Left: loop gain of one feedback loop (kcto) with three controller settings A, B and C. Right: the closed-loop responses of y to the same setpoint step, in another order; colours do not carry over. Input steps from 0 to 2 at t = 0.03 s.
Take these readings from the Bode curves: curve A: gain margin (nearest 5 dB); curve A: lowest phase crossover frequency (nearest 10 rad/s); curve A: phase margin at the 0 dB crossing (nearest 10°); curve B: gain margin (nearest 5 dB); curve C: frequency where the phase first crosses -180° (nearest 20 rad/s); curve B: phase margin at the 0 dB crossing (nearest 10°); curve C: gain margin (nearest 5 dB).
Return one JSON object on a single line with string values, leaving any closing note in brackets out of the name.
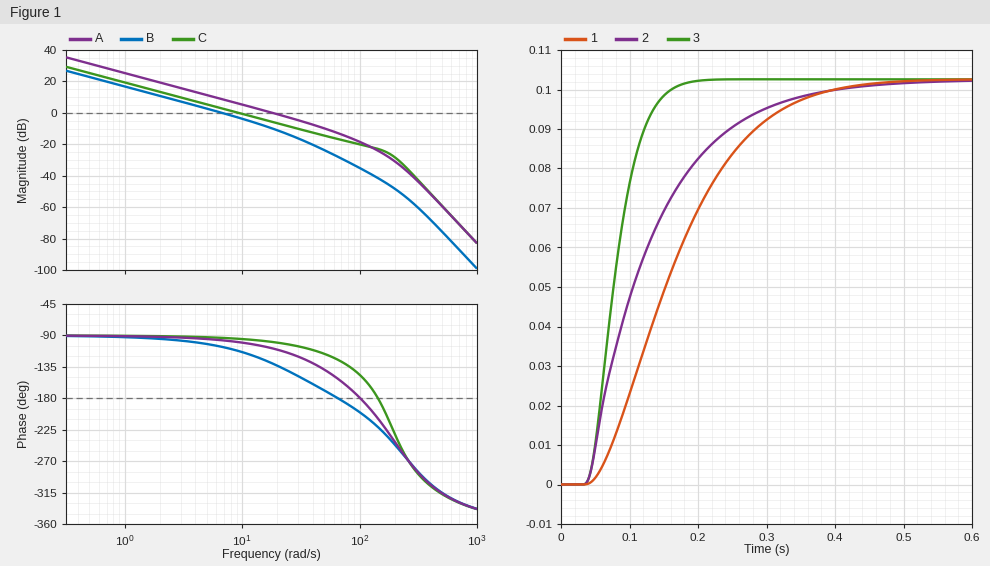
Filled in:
{"curve A: gain margin": "20 dB", "curve A: lowest phase crossover frequency": "100 rad/s", "curve A: phase margin at the 0 dB crossing": "70°", "curve B: gain margin": "30 dB", "curve C: frequency where the phase first crosses -180°": "140 rad/s", "curve B: phase margin at the 0 dB crossing": "70°", "curve C: gain margin": "25 dB"}
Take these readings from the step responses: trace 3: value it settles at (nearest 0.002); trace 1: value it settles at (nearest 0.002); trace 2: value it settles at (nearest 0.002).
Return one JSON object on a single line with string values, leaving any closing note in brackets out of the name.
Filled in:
{"trace 3: value it settles at": "0.102", "trace 1: value it settles at": "0.102", "trace 2: value it settles at": "0.102"}
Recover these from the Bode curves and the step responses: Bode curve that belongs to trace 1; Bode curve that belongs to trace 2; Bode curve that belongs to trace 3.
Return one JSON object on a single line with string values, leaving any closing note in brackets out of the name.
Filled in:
{"Bode curve that belongs to trace 1": "B", "Bode curve that belongs to trace 2": "C", "Bode curve that belongs to trace 3": "A"}
